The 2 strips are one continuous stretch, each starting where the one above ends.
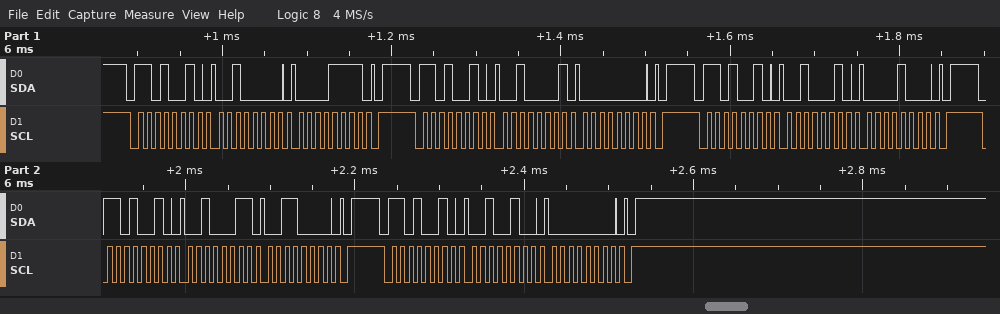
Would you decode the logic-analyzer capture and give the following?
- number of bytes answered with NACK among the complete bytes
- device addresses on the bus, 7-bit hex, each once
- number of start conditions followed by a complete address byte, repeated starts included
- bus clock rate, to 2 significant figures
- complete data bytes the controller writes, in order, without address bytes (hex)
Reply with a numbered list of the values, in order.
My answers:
1. 0
2. 0x69
3. 5
4. 100 kHz
5. 20 0F 21 00 22 08 23 30 24 00
